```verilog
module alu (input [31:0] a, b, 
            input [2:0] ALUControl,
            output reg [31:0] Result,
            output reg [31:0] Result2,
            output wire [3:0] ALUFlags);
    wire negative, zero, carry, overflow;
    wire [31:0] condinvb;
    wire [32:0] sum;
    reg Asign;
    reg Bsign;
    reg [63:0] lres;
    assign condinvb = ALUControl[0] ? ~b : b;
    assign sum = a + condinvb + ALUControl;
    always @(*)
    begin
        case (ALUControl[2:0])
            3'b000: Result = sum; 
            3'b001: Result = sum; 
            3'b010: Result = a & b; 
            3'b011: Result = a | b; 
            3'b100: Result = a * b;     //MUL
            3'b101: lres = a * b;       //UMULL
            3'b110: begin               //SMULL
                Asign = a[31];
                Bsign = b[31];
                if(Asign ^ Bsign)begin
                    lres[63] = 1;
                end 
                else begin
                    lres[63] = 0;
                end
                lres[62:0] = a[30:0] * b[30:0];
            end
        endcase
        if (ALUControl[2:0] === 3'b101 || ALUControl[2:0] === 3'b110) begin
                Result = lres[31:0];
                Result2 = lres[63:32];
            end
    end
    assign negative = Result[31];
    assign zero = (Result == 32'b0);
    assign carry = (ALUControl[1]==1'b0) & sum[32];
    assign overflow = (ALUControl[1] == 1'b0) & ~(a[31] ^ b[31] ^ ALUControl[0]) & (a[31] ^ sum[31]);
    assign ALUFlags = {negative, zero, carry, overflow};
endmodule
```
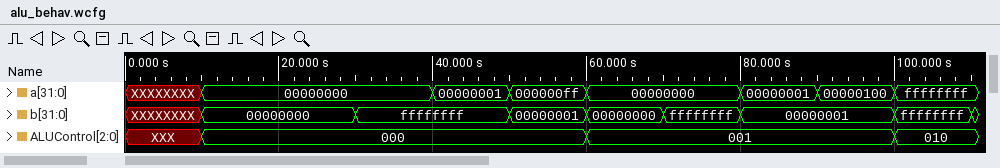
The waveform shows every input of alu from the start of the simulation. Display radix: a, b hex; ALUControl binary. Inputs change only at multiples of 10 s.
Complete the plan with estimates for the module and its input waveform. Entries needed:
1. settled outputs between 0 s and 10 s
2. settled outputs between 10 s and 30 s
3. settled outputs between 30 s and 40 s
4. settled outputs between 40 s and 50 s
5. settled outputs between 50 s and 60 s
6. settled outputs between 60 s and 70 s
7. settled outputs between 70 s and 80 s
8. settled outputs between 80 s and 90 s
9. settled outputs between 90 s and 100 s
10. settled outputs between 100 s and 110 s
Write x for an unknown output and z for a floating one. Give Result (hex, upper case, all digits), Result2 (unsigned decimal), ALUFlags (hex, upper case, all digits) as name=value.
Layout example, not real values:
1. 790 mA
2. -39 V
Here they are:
1. Result=x, Result2=x, ALUFlags=x
2. Result=00000000, Result2=x, ALUFlags=4
3. Result=FFFFFFFF, Result2=x, ALUFlags=8
4. Result=00000000, Result2=x, ALUFlags=6
5. Result=00000100, Result2=x, ALUFlags=0
6. Result=00000000, Result2=x, ALUFlags=6
7. Result=00000001, Result2=x, ALUFlags=0
8. Result=00000000, Result2=x, ALUFlags=6
9. Result=000000FF, Result2=x, ALUFlags=2
10. Result=FFFFFFFF, Result2=x, ALUFlags=8
